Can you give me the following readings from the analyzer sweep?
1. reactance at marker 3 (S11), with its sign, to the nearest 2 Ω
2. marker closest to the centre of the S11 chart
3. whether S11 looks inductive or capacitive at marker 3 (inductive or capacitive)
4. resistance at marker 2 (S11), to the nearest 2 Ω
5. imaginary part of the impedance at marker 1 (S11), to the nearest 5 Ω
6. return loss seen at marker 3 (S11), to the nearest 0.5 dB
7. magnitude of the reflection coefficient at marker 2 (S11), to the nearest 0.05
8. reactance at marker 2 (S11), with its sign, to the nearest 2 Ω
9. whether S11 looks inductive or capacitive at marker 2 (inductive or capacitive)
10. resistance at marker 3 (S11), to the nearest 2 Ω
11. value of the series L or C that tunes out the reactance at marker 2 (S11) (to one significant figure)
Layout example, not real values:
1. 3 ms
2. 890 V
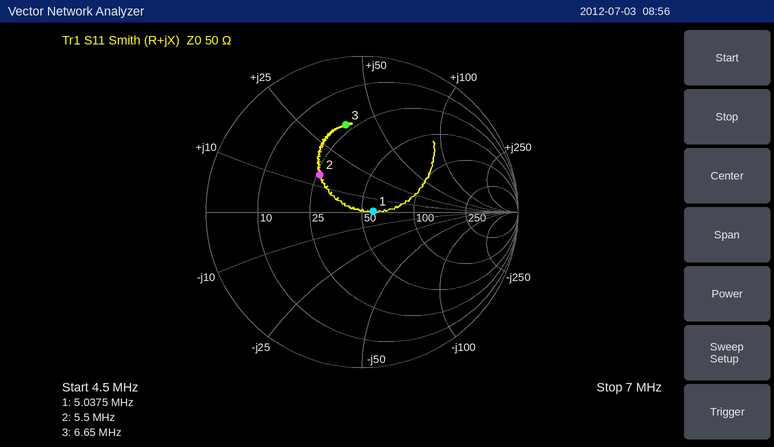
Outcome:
1. +36 Ω
2. marker 1
3. inductive
4. 26 Ω
5. 0 Ω
6. 5.0 dB
7. 0.35
8. +14 Ω
9. inductive
10. 22 Ω
11. 2 nF
